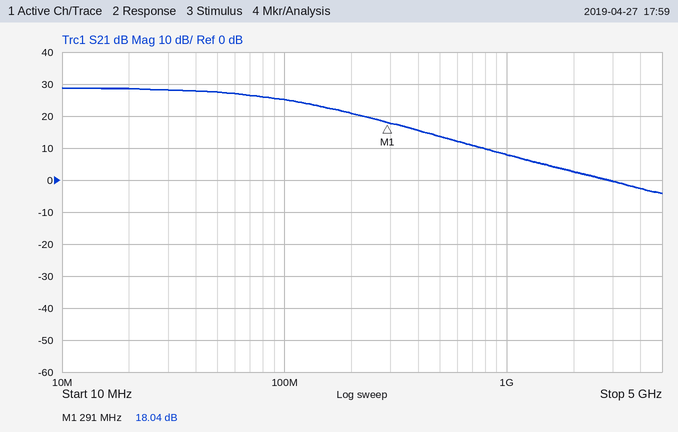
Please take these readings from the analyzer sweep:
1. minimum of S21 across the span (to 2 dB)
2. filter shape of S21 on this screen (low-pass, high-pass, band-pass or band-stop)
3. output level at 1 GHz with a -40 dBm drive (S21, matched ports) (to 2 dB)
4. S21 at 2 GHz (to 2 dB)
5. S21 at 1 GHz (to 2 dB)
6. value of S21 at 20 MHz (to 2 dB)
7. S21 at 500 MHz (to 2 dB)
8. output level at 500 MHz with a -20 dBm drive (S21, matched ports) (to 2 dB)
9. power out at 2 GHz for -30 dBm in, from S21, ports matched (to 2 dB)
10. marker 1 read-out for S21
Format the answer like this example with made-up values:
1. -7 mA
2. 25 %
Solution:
1. -4 dB
2. low-pass
3. -32 dBm
4. 2 dB
5. 8 dB
6. 28 dB
7. 14 dB
8. -6 dBm
9. -28 dBm
10. 18.04 dB
